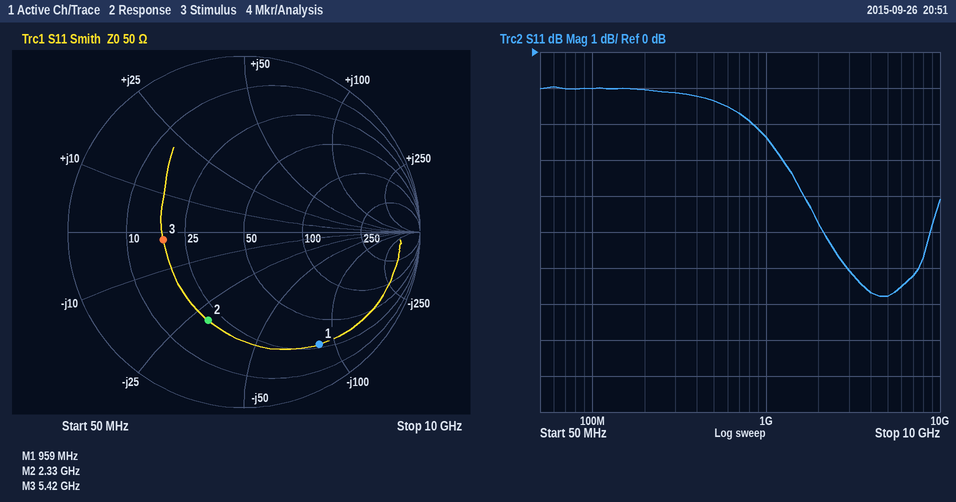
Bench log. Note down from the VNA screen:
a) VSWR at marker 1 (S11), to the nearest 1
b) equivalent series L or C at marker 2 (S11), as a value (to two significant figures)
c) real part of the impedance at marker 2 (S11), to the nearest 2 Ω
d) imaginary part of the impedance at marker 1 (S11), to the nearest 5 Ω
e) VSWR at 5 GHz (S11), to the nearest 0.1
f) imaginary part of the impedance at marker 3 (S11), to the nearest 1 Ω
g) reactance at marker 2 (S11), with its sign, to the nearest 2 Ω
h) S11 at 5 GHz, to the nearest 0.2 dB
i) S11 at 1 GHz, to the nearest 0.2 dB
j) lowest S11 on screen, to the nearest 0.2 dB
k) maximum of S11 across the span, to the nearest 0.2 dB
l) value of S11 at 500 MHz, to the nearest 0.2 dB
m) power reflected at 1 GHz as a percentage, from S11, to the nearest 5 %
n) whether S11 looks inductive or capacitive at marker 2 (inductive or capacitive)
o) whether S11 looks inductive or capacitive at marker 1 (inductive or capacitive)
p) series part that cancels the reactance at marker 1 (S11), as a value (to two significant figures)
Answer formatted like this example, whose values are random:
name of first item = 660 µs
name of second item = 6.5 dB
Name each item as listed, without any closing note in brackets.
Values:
VSWR at marker 1 (S11), to the nearest 1 = 8
equivalent series L or C at marker 2 (S11), as a value = 2.3 pF
real part of the impedance at marker 2 (S11), to the nearest 2 Ω = 20 Ω
imaginary part of the impedance at marker 1 (S11), to the nearest 5 Ω = -85 Ω
VSWR at 5 GHz (S11), to the nearest 0.1 = 2.7
imaginary part of the impedance at marker 3 (S11), to the nearest 1 Ω = -2 Ω
reactance at marker 2 (S11), with its sign, to the nearest 2 Ω = -30 Ω
S11 at 5 GHz, to the nearest 0.2 dB = -6.8 dB
S11 at 1 GHz, to the nearest 0.2 dB = -2.4 dB
lowest S11 on screen, to the nearest 0.2 dB = -6.8 dB
maximum of S11 across the span, to the nearest 0.2 dB = -1.0 dB
value of S11 at 500 MHz, to the nearest 0.2 dB = -1.4 dB
power reflected at 1 GHz as a percentage, from S11, to the nearest 5 % = 60 %
whether S11 looks inductive or capacitive at marker 2 = capacitive
whether S11 looks inductive or capacitive at marker 1 = capacitive
series part that cancels the reactance at marker 1 (S11), as a value = 14 nH
